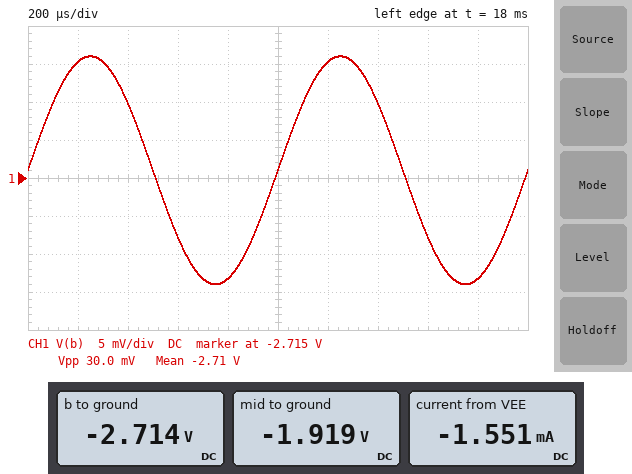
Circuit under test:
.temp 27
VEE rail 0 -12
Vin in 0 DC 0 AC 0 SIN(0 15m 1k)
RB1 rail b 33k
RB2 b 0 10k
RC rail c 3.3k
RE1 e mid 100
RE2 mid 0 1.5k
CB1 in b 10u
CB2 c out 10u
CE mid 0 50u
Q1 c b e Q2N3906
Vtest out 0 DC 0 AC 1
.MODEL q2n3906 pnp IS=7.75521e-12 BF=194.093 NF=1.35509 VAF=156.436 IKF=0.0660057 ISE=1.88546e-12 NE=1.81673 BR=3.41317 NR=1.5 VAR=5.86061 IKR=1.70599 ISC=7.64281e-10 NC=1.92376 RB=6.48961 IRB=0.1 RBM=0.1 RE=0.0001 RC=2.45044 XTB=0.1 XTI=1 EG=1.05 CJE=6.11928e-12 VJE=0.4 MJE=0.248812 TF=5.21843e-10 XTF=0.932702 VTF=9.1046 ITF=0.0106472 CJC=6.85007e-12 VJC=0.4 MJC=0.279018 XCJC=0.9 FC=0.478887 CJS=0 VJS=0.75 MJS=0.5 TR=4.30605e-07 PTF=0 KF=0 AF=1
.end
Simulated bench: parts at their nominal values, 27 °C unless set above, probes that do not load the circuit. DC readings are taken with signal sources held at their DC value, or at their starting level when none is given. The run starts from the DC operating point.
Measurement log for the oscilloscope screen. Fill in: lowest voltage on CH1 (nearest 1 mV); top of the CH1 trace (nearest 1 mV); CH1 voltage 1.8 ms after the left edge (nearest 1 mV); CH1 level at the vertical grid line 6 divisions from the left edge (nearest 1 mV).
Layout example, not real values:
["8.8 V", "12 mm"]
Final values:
["-2.729 V", "-2.699 V", "-2.728 V", "-2.700 V"]
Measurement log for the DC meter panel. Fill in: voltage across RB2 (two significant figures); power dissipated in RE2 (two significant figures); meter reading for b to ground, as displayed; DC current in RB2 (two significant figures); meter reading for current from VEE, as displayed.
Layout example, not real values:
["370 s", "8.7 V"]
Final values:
["2.7 V", "2.5 mW", "-2.714 V", "270 µA", "-1.551 mA"]
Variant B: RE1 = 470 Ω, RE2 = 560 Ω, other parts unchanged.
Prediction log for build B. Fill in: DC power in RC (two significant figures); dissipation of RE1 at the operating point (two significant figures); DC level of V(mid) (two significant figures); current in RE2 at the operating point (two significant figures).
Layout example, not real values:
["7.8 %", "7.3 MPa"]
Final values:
["12 mW", "1.8 mW", "-1.1 V", "1.9 mA"]
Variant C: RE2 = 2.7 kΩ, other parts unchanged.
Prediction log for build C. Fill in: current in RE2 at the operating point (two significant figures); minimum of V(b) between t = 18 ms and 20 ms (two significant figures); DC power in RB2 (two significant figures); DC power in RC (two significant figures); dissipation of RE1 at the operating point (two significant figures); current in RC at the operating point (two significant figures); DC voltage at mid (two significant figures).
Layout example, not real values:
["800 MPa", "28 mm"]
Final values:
["750 µA", "-2.8 V", "750 µW", "1.8 mW", "56 µW", "740 µA", "-2.0 V"]
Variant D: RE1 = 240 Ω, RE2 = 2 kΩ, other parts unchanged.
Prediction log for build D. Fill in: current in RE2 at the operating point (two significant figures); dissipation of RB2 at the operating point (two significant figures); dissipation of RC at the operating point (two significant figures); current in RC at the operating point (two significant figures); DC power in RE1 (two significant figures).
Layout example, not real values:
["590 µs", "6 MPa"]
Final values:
["930 µA", "750 µW", "2.8 mW", "920 µA", "210 µW"]
